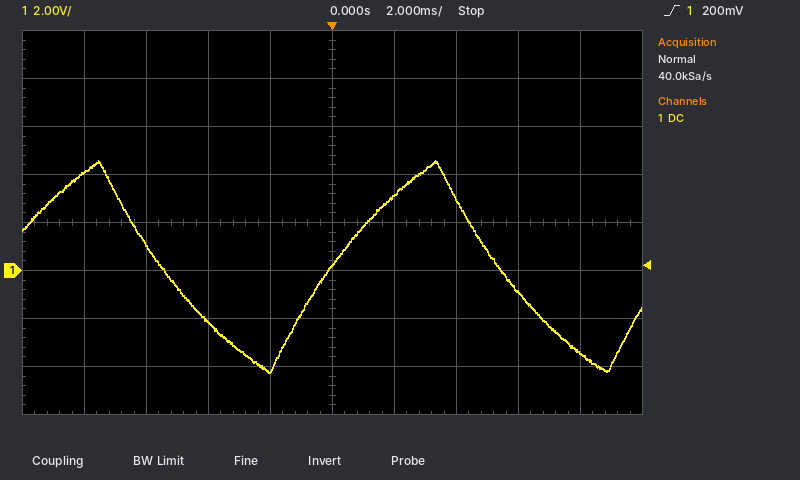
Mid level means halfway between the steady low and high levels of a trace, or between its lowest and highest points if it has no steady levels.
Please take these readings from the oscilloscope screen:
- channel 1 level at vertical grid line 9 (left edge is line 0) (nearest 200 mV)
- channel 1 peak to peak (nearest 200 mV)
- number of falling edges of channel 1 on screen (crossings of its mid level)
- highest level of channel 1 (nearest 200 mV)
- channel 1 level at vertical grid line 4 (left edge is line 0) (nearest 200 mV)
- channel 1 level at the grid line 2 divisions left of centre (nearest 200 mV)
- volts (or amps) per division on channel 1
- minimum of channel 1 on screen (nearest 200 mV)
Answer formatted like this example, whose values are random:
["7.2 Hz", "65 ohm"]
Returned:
["-3.4 V", "8.8 V", "2", "4.6 V", "-4.2 V", "-2.2 V", "2 V", "-4.2 V"]
